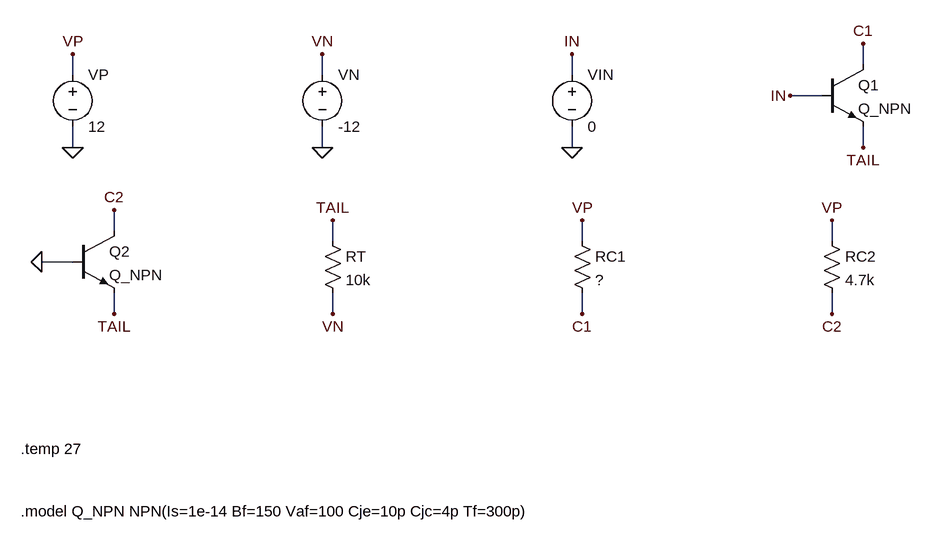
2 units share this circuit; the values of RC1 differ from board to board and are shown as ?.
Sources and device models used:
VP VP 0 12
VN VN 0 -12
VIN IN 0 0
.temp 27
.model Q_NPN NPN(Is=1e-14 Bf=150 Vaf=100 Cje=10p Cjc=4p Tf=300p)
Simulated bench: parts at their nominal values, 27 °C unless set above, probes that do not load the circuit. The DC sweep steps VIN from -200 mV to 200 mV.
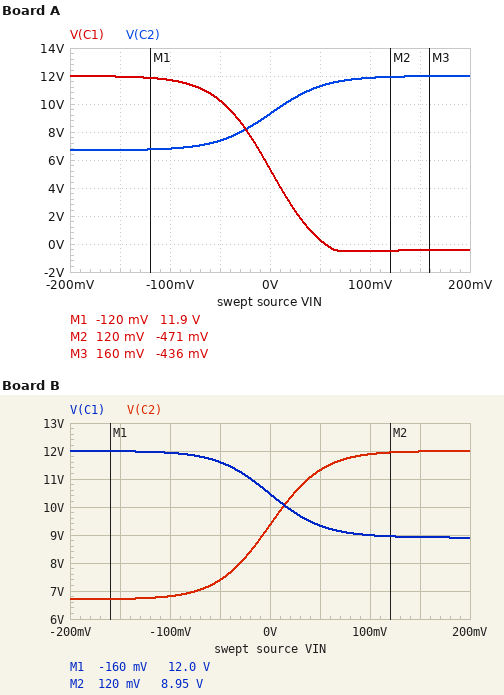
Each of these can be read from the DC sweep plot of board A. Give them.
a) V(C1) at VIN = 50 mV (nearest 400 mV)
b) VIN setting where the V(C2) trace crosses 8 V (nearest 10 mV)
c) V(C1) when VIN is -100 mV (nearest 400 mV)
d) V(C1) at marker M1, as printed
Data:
400 mV
-30 mV
11.6 V
11.9 V
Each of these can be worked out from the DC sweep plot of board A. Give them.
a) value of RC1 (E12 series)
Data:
12 kΩ
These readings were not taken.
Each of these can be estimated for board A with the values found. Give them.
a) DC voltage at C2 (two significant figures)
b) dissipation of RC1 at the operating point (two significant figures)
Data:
9.3 V
3.7 mW
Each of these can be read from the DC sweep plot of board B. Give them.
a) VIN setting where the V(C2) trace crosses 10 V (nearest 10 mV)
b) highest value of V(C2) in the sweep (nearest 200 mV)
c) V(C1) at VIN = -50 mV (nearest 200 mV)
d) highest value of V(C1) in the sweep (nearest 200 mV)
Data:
10 mV
12.0 V
11.6 V
12.0 V
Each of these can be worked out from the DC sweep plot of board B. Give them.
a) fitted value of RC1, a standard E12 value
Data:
2.7 kΩ
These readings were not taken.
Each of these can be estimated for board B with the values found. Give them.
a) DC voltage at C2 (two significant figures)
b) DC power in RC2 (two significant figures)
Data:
9.4 V
1.5 mW
